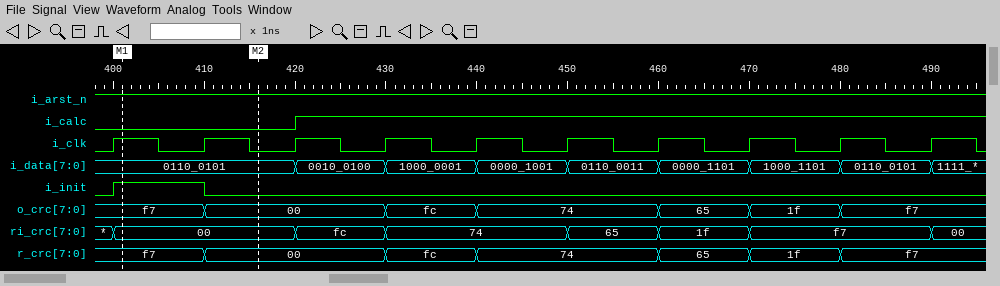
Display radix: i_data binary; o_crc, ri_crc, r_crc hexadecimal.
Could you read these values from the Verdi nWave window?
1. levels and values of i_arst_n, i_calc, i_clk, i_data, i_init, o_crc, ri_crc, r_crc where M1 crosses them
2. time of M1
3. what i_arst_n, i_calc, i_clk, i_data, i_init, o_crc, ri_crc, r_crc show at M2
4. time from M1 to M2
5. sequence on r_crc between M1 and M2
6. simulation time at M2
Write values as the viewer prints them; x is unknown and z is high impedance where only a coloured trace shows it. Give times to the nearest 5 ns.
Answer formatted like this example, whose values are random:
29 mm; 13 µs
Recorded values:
i_arst_n=1, i_calc=0, i_clk=1, i_data=0110_0101, i_init=1, o_crc=f7, ri_crc=00, r_crc=f7; 400 ns; i_arst_n=1, i_calc=0, i_clk=0, i_data=0110_0101, i_init=0, o_crc=00, ri_crc=00, r_crc=00; 15 ns; f7, 00; 415 ns
